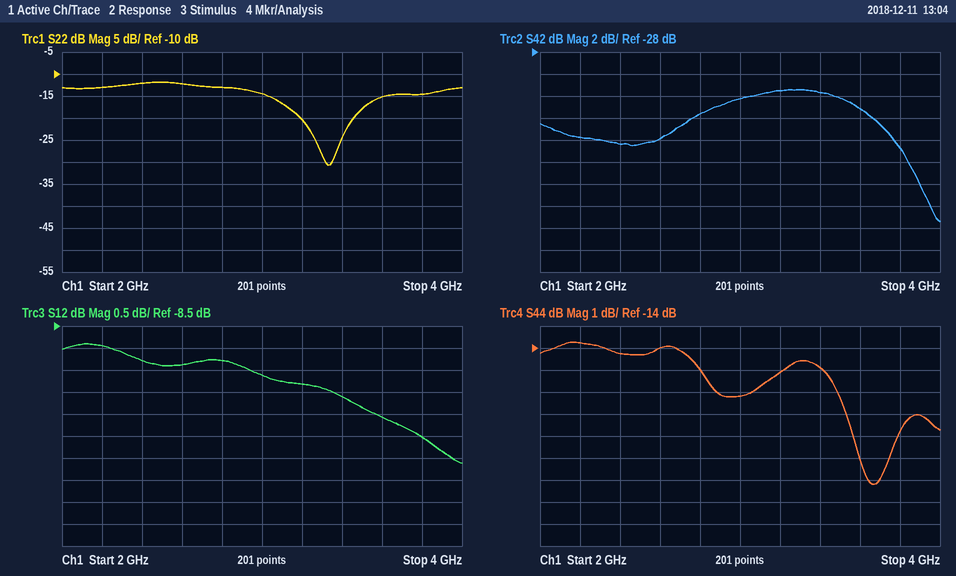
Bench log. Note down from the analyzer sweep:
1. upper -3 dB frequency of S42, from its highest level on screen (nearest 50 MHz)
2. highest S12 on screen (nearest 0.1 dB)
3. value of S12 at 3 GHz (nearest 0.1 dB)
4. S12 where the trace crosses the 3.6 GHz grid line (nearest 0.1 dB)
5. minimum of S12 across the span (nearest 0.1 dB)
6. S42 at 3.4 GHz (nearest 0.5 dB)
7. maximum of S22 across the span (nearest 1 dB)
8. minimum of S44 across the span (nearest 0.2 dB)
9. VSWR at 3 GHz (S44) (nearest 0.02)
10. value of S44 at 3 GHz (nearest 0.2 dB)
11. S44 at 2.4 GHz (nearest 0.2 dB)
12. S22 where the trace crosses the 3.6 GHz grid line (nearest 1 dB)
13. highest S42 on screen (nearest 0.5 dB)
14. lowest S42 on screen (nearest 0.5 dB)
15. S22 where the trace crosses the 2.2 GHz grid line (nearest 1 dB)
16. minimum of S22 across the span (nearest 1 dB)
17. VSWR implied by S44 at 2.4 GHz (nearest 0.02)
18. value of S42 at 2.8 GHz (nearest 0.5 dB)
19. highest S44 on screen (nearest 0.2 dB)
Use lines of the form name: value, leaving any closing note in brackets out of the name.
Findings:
upper -3 dB frequency of S42, from its highest level on screen: 3.70 GHz
highest S12 on screen: -8.9 dB
value of S12 at 3 GHz: -9.6 dB
S12 where the trace crosses the 3.6 GHz grid line: -10.6 dB
minimum of S12 across the span: -11.6 dB
S42 at 3.4 GHz: -31.5 dB
maximum of S22 across the span: -12 dB
minimum of S44 across the span: -20.2 dB
VSWR at 3 GHz (S44): 1.36
value of S44 at 3 GHz: -16.2 dB
S44 at 2.4 GHz: -14.2 dB
S22 where the trace crosses the 3.6 GHz grid line: -15 dB
highest S42 on screen: -31.5 dB
lowest S42 on screen: -43.5 dB
S22 where the trace crosses the 2.2 GHz grid line: -13 dB
minimum of S22 across the span: -31 dB
VSWR implied by S44 at 2.4 GHz: 1.48
value of S42 at 2.8 GHz: -33.5 dB
highest S44 on screen: -13.8 dB
